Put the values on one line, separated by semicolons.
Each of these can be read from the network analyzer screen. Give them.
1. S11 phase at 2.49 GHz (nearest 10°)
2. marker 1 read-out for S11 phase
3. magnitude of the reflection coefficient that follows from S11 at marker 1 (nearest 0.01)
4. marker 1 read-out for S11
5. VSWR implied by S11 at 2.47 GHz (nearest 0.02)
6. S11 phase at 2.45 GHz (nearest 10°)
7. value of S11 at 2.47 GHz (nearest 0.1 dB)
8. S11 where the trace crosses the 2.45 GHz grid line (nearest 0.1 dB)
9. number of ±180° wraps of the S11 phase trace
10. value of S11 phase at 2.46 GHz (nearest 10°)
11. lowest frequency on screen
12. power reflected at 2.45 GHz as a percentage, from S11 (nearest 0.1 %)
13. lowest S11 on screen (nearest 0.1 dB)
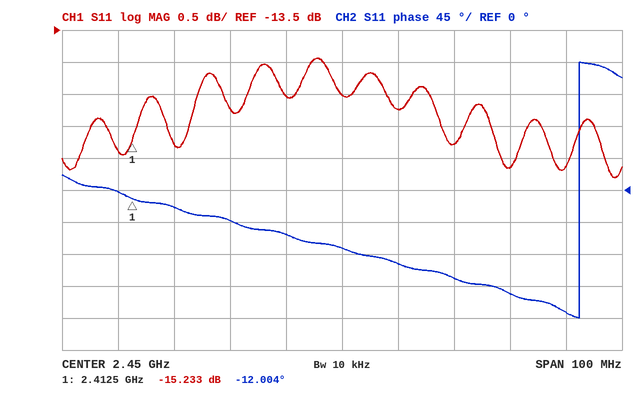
-170°; -12.004°; 0.17; -15.233 dB; 1.42; -80°; -15.3 dB; -14.5 dB; 1; -100°; 2.4 GHz; 3.5 %; -15.8 dB
